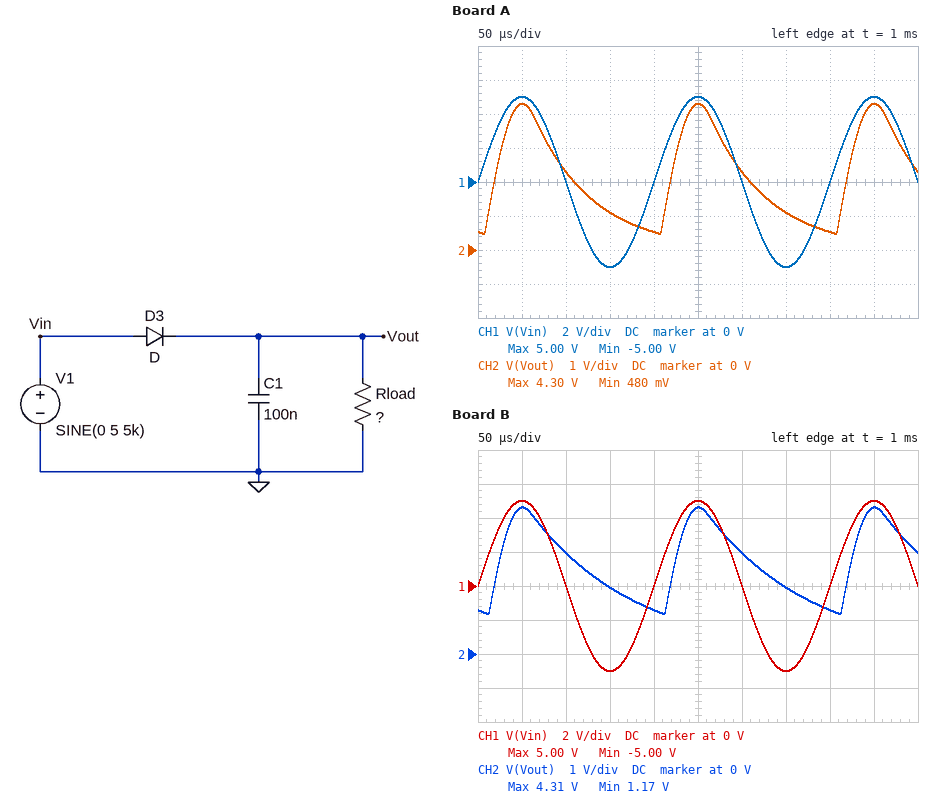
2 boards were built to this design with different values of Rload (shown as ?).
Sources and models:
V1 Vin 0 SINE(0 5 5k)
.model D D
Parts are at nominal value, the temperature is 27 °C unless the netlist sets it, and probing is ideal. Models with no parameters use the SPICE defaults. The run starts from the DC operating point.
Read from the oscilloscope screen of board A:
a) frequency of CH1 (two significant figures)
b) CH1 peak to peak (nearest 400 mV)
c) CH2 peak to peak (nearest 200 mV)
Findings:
5.0 kHz
10.0 V
3.8 V
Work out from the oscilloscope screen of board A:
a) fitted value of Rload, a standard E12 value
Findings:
680 Ω
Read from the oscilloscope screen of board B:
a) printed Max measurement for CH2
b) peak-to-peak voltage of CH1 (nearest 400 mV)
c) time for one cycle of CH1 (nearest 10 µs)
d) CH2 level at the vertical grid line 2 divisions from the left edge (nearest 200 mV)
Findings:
4.31 V
10.0 V
200 µs
3.0 V
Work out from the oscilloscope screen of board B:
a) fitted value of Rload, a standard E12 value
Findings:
1.2 kΩ
